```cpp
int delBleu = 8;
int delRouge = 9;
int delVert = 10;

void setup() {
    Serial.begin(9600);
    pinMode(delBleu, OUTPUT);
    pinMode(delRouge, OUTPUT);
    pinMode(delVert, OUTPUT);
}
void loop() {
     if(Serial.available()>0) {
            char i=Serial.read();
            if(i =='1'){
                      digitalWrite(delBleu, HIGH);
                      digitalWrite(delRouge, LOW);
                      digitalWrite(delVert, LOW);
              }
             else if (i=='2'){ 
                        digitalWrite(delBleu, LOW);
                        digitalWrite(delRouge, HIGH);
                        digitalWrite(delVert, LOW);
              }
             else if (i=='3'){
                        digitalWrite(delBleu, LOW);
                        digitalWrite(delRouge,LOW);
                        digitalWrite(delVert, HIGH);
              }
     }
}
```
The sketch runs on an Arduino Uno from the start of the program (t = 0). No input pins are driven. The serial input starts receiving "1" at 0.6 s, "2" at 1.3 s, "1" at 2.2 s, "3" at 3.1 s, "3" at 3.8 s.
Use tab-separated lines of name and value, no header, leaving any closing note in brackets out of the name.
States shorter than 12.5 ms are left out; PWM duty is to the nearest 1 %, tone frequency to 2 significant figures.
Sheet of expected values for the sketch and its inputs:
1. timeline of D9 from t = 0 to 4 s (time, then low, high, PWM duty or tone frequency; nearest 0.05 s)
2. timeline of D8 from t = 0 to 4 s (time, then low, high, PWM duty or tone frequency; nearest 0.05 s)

timeline of D9 from t = 0 to 4 s	0 s low; 1.3 s high; 2.2 s low
timeline of D8 from t = 0 to 4 s	0 s low; 0.6 s high; 1.3 s low; 2.2 s high; 3.1 s low
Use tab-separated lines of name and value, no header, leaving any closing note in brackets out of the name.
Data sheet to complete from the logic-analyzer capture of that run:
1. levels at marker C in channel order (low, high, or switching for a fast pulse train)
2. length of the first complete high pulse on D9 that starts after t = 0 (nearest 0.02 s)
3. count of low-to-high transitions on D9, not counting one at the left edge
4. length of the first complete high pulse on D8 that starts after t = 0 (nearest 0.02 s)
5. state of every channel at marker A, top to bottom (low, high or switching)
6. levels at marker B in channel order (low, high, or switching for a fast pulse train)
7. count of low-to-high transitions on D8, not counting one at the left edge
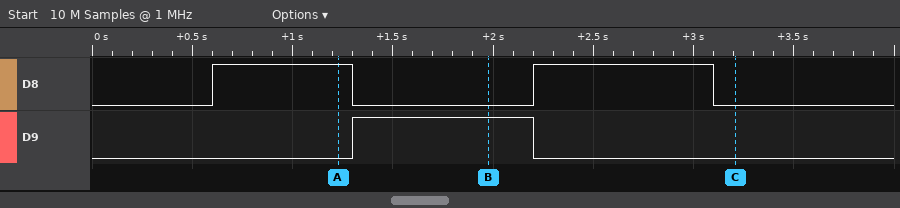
levels at marker C in channel order	D8 low, D9 low
length of the first complete high pulse on D9 that starts after t = 0	0.90 s
count of low-to-high transitions on D9, not counting one at the left edge	1
length of the first complete high pulse on D8 that starts after t = 0	0.70 s
state of every channel at marker A, top to bottom	D8 high, D9 low
levels at marker B in channel order	D8 low, D9 high
count of low-to-high transitions on D8, not counting one at the left edge	2
